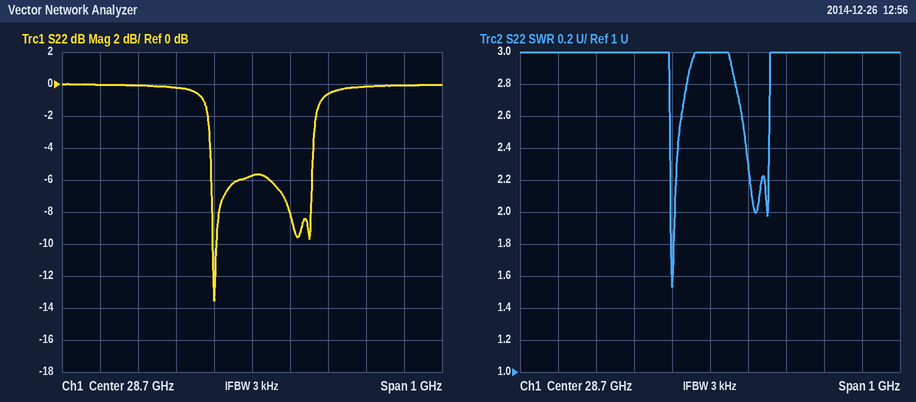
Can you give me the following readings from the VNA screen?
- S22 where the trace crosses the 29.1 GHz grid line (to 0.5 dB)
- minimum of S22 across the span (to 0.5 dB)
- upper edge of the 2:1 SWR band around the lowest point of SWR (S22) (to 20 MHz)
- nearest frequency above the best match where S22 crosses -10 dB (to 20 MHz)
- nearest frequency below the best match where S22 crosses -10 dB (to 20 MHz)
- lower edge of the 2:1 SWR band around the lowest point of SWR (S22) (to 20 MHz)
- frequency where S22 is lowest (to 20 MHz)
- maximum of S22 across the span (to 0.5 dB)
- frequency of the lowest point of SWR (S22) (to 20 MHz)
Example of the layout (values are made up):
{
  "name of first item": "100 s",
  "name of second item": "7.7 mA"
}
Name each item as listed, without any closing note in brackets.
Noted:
{
  "S22 where the trace crosses the 29.1 GHz grid line": "0.0 dB",
  "minimum of S22 across the span": "-13.5 dB",
  "upper edge of the 2:1 SWR band around the lowest point of SWR (S22)": "28.60 GHz",
  "nearest frequency above the best match where S22 crosses -10 dB": "28.60 GHz",
  "nearest frequency below the best match where S22 crosses -10 dB": "28.60 GHz",
  "lower edge of the 2:1 SWR band around the lowest point of SWR (S22)": "28.60 GHz",
  "frequency where S22 is lowest": "28.60 GHz",
  "maximum of S22 across the span": "0.0 dB",
  "frequency of the lowest point of SWR (S22)": "28.60 GHz"
}
